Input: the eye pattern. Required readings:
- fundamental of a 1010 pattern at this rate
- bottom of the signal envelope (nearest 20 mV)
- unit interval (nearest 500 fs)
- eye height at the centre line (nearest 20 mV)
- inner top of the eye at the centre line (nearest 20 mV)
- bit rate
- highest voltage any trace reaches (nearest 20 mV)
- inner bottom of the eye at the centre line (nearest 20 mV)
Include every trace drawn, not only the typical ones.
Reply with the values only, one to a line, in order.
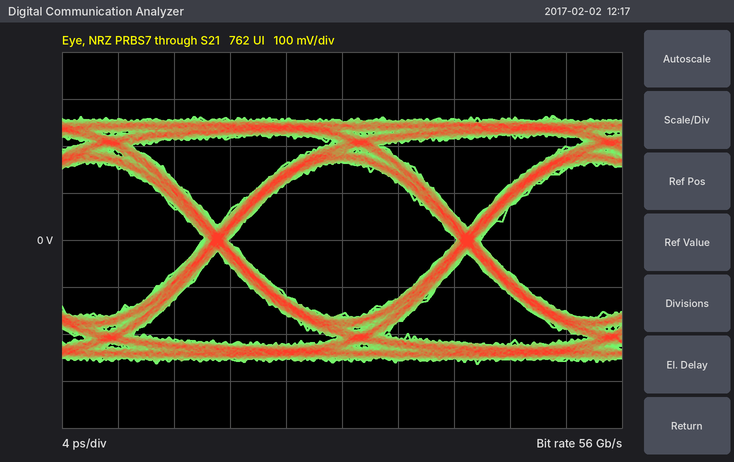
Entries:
28 GHz
-260 mV
18.0 ps
320 mV
160 mV
56 Gb/s
260 mV
-160 mV
